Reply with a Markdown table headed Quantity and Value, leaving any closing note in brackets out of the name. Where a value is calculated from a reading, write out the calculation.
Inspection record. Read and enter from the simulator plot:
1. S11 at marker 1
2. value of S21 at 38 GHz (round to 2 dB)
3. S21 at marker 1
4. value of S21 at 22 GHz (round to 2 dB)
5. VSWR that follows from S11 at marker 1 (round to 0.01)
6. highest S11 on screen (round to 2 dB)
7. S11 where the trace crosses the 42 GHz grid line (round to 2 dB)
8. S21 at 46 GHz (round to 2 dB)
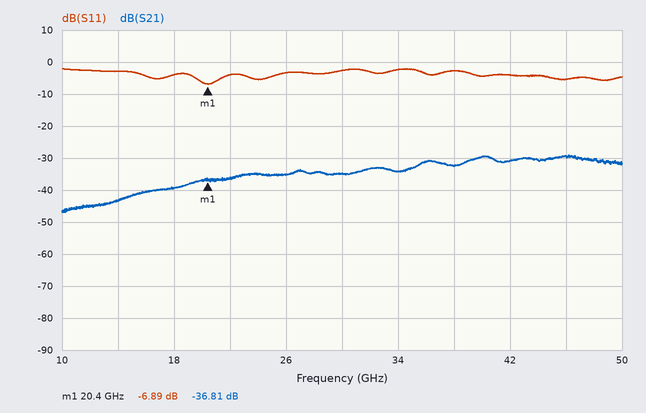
| Quantity | Value |
|---|---|
| S11 at marker 1 | -6.89 dB |
| value of S21 at 38 GHz | -32 dB |
| S21 at marker 1 | -36.81 dB |
| value of S21 at 22 GHz | -36 dB |
| VSWR that follows from S11 at marker 1 | (1 + 0.4524)/(1 − 0.4524) ≈ 2.65 |
| highest S11 on screen | -2 dB |
| S11 where the trace crosses the 42 GHz grid line | -4 dB |
| S21 at 46 GHz | -30 dB |
